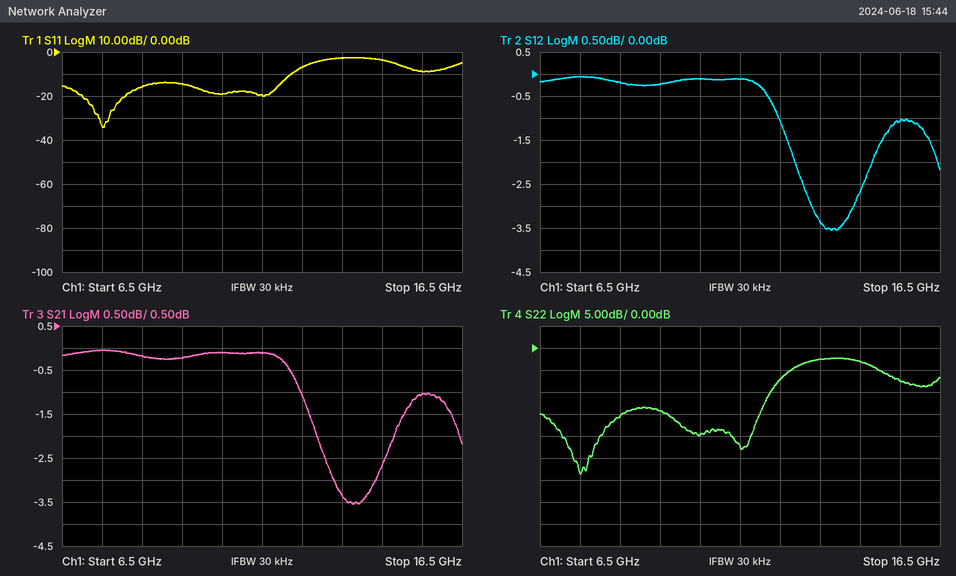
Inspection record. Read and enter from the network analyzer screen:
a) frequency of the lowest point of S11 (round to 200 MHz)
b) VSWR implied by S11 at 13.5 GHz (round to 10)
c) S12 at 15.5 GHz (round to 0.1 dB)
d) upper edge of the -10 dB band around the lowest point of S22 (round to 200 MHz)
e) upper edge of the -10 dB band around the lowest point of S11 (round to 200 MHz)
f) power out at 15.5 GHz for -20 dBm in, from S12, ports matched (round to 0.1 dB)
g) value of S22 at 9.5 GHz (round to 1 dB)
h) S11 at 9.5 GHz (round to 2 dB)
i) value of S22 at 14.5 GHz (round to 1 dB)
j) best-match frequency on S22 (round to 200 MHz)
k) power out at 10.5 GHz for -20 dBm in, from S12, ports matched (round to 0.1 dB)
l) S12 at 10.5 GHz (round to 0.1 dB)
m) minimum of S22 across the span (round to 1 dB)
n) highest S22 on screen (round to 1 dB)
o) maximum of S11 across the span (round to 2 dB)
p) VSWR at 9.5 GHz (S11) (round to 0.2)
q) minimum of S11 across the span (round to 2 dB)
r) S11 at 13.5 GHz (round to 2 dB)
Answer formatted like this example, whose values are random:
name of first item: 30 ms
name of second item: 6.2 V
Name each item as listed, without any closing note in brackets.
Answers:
frequency of the lowest point of S11: 7.6 GHz
VSWR implied by S11 at 13.5 GHz: 10
S12 at 15.5 GHz: -1.1 dB
upper edge of the -10 dB band around the lowest point of S22: 12.2 GHz
upper edge of the -10 dB band around the lowest point of S11: 12.2 GHz
power out at 15.5 GHz for -20 dBm in, from S12, ports matched: -21.1 dBm
value of S22 at 9.5 GHz: -14 dB
S11 at 9.5 GHz: -14 dB
value of S22 at 14.5 GHz: -3 dB
best-match frequency on S22: 7.6 GHz
power out at 10.5 GHz for -20 dBm in, from S12, ports matched: -20.1 dBm
S12 at 10.5 GHz: -0.1 dB
minimum of S22 across the span: -29 dB
highest S22 on screen: -2 dB
maximum of S11 across the span: -2 dB
VSWR at 9.5 GHz (S11): 1.4
minimum of S11 across the span: -34 dB
S11 at 13.5 GHz: -2 dB
